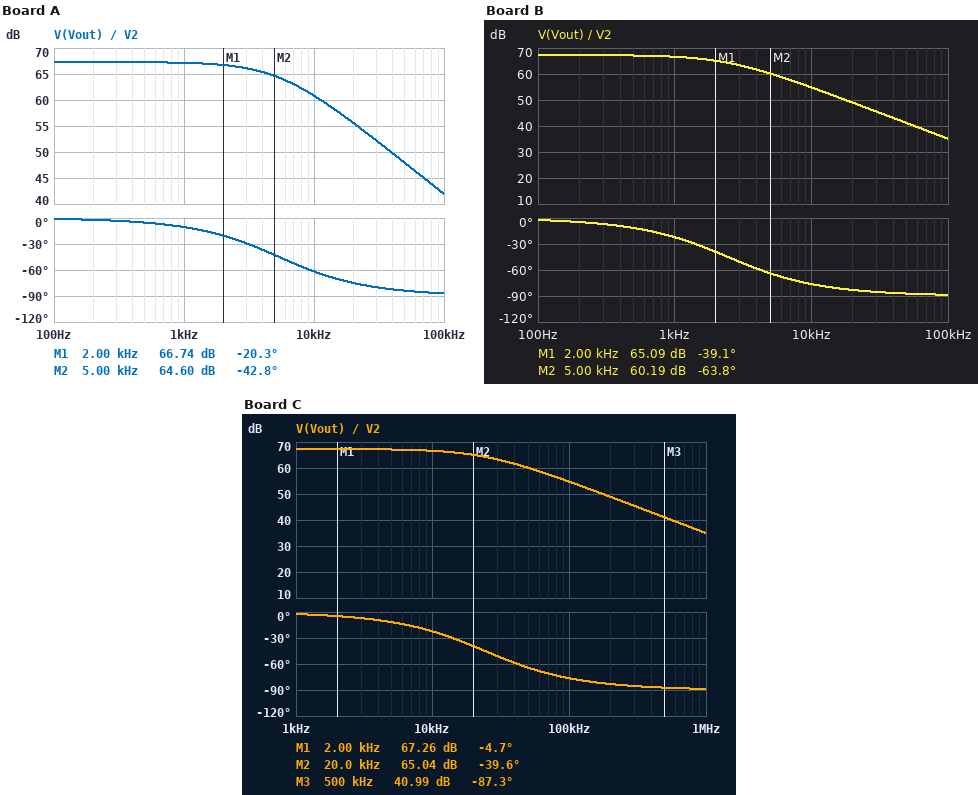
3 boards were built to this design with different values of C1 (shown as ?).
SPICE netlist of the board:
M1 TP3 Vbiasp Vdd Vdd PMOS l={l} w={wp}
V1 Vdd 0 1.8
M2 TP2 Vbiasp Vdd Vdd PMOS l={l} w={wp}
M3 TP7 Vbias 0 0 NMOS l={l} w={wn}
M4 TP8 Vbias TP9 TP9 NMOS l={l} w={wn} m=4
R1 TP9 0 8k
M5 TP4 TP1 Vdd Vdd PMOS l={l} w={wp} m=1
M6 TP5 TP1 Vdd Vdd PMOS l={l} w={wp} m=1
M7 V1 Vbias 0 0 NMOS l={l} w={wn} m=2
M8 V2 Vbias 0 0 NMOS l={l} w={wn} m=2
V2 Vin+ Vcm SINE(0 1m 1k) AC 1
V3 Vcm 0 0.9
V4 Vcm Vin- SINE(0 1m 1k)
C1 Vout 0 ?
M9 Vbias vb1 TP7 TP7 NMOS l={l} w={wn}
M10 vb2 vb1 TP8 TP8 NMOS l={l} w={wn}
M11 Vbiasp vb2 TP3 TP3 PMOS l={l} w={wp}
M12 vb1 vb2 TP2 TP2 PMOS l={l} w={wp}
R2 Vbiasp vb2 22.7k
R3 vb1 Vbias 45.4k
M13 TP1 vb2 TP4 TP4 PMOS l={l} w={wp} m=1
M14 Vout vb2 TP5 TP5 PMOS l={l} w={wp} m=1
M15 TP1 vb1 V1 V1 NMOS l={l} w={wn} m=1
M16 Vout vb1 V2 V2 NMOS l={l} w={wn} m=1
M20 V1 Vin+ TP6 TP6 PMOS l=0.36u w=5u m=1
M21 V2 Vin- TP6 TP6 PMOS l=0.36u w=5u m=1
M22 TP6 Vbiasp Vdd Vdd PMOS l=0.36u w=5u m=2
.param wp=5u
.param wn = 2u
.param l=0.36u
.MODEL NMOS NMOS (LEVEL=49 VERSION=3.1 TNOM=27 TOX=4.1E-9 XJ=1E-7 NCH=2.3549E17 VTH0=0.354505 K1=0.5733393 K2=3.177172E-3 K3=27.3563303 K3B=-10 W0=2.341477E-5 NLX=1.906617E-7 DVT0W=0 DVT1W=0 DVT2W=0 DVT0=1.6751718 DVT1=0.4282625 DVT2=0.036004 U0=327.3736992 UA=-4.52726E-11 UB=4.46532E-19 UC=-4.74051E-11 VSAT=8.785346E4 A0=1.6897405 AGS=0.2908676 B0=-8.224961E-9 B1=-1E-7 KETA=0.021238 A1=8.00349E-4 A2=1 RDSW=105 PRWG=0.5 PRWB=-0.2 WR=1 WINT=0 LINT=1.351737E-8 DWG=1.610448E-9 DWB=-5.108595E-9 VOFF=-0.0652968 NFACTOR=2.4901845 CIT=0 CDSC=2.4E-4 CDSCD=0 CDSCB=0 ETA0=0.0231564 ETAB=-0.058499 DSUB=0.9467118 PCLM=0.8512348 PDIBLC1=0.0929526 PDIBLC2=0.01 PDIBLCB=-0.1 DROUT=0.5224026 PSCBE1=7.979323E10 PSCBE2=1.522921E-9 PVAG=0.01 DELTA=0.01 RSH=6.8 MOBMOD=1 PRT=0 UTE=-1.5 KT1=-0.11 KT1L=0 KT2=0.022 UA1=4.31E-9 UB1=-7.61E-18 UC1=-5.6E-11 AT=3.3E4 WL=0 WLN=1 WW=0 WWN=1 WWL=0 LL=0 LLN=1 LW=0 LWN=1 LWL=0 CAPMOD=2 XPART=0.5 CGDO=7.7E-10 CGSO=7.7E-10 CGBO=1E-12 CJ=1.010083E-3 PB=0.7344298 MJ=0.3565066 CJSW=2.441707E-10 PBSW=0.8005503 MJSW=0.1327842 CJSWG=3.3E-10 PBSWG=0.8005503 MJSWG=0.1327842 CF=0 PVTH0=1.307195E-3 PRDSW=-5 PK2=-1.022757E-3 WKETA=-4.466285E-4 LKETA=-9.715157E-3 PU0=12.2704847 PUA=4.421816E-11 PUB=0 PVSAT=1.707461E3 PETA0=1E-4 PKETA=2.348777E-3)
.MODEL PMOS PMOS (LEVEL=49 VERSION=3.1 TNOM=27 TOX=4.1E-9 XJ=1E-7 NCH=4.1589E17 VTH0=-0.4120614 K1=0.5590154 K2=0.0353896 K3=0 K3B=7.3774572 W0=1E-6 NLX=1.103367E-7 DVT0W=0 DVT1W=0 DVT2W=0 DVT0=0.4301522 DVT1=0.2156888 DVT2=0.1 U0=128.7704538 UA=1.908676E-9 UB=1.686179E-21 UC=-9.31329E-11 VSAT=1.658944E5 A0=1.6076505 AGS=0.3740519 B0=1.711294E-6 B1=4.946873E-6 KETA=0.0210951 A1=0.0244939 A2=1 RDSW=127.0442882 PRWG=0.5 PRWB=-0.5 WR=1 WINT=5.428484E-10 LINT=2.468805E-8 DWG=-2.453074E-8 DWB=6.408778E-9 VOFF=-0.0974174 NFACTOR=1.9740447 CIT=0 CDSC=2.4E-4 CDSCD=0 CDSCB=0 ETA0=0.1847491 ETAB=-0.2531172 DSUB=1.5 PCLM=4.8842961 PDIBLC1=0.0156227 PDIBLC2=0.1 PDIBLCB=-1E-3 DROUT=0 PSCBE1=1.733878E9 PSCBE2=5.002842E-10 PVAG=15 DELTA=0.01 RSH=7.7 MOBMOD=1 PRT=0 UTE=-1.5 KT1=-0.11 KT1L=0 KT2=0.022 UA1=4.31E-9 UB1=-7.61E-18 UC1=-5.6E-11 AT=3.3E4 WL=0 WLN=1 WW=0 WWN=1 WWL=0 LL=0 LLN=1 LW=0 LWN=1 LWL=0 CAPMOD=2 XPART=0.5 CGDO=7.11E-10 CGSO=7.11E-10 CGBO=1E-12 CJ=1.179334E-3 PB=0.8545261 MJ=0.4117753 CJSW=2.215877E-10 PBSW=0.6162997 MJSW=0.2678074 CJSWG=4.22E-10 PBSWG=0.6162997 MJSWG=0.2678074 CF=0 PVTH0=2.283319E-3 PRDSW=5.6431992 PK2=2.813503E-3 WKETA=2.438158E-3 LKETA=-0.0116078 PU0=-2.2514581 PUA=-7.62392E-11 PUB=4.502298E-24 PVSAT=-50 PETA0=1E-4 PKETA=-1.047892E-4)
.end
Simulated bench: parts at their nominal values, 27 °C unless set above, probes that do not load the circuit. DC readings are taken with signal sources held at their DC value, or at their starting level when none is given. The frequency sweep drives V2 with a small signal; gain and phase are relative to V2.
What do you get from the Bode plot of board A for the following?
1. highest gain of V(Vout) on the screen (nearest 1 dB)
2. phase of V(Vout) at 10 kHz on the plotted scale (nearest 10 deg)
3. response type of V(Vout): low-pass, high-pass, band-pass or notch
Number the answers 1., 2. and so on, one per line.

1. 67 dB
2. -60 deg
3. low-pass
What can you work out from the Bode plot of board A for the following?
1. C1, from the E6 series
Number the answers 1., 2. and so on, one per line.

1. 1.5 pF
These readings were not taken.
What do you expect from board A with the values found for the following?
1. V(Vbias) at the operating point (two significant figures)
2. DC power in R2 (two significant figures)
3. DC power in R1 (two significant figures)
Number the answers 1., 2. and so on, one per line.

1. 600 mV
2. 1.8 µW
3. 650 nW
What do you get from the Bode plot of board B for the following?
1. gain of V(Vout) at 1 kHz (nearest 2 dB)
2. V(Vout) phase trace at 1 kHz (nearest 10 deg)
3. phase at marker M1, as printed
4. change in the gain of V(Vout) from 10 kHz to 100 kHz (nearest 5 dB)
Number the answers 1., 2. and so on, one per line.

1. 66 dB
2. -20 deg
3. -39.1 deg
4. -20 dB
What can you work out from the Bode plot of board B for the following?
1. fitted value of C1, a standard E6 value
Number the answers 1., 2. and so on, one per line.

1. 3.3 pF
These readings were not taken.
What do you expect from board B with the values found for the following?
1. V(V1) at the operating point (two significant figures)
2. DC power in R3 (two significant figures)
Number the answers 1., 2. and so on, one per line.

1. 410 mV
2. 3.7 µW
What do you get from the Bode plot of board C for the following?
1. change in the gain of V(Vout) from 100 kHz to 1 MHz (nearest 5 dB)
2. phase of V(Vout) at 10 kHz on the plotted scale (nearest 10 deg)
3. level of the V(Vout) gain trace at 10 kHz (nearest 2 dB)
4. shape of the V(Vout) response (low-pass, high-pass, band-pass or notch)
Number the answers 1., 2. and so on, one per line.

1. -20 dB
2. -20 deg
3. 66 dB
4. low-pass
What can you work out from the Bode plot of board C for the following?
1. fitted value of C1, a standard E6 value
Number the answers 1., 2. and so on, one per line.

1. 330 fF
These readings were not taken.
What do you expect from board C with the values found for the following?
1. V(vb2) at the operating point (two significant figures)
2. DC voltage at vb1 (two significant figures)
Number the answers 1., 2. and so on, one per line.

1. 990 mV
2. 1.0 V
